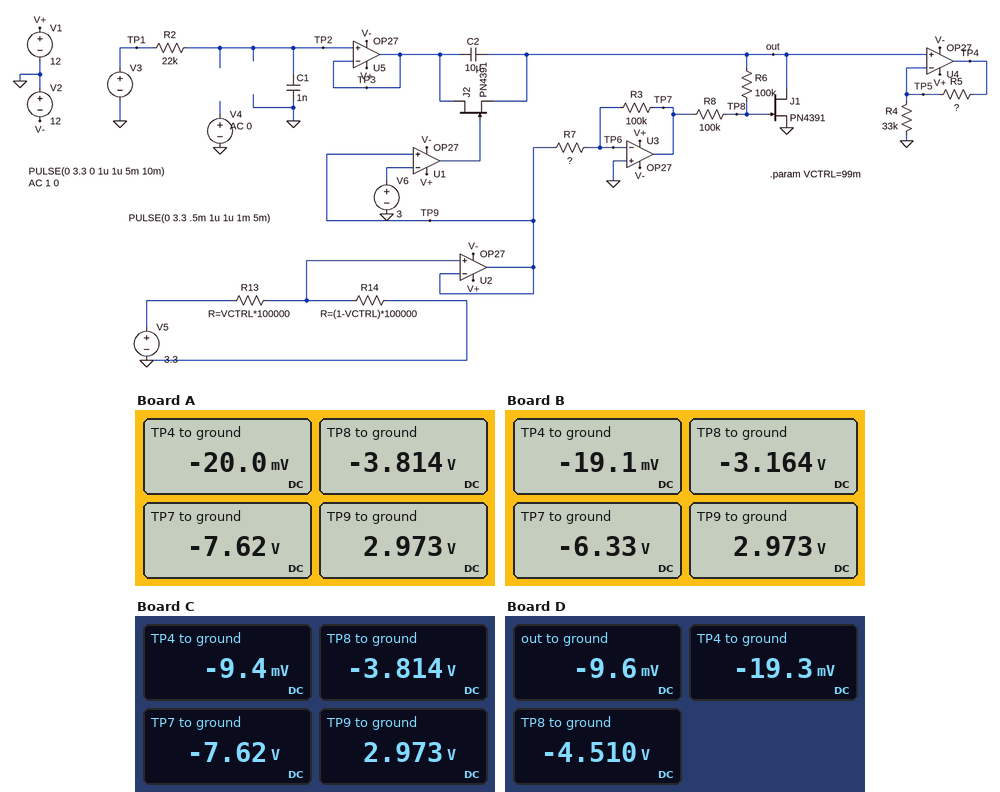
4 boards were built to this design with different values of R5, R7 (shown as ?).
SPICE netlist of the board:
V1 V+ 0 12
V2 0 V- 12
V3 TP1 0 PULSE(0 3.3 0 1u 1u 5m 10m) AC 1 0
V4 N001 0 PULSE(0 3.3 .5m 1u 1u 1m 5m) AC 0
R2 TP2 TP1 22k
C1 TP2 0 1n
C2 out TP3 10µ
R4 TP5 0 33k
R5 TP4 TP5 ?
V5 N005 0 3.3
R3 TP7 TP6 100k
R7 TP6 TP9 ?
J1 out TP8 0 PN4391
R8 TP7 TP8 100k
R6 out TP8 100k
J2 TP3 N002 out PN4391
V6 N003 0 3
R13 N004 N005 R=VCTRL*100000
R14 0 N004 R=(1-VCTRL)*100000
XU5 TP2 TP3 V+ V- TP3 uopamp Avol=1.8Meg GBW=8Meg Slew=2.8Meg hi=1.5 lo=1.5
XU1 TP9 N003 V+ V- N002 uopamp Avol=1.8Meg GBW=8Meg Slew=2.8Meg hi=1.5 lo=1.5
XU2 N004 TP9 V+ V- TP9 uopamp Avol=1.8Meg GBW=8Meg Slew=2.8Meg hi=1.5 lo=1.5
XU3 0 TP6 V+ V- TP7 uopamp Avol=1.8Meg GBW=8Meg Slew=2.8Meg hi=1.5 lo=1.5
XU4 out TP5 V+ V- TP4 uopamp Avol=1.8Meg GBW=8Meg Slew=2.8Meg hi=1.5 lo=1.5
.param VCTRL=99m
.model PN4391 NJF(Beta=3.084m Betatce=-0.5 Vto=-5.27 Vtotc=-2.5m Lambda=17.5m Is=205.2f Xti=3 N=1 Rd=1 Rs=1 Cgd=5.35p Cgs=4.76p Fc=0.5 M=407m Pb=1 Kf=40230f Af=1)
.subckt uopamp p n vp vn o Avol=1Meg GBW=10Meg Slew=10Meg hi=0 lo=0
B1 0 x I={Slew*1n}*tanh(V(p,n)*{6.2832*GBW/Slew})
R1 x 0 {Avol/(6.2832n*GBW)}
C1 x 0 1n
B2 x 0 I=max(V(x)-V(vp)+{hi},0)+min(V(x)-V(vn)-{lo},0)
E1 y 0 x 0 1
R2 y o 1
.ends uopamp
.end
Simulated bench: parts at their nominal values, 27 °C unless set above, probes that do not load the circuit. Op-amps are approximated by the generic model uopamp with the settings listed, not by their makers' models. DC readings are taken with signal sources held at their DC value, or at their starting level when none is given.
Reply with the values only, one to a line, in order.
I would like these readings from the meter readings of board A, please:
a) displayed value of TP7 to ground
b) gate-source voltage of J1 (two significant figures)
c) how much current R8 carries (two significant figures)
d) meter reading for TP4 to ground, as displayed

-7.62 V
-3.8 V
38 µA
-20.0 mV
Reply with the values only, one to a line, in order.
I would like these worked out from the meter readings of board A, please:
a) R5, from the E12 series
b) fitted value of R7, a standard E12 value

120 kΩ
39 kΩ
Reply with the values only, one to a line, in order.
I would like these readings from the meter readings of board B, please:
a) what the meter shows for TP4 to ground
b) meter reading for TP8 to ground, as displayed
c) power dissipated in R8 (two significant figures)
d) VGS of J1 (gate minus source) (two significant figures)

-19.1 mV
-3.164 V
100 µW
-3.2 V
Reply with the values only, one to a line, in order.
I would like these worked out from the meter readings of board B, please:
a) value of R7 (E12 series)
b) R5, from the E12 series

47 kΩ
220 kΩ
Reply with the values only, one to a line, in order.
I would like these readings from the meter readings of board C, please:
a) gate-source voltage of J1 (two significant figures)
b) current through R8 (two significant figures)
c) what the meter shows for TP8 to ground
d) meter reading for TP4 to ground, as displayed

-3.8 V
38 µA
-3.814 V
-9.4 mV
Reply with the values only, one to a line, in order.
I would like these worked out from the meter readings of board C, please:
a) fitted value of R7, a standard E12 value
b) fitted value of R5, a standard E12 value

39 kΩ
39 kΩ
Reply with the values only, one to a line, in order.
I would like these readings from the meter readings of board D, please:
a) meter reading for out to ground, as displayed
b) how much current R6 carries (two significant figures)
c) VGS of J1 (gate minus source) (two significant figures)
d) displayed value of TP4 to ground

-9.6 mV
45 µA
-4.5 V
-19.3 mV
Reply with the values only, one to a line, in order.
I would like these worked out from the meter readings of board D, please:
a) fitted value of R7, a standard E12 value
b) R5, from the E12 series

33 kΩ
33 kΩ
